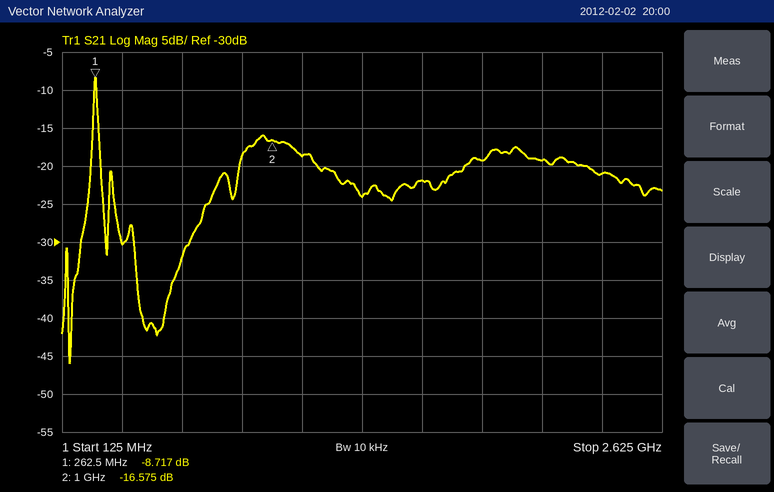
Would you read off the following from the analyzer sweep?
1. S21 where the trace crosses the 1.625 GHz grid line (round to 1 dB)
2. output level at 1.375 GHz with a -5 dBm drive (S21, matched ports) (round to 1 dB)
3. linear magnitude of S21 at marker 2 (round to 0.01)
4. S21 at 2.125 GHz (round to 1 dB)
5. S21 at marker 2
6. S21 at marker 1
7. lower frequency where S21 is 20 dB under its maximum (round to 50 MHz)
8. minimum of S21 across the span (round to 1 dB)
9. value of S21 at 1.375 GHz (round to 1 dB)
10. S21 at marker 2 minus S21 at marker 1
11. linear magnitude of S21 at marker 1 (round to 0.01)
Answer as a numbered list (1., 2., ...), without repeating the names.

1. -22 dB
2. -29 dBm
3. 0.15
4. -19 dB
5. -16.575 dB
6. -8.717 dB
7. 200 MHz
8. -46 dB
9. -24 dB
10. -7.858 dB
11. 0.37
